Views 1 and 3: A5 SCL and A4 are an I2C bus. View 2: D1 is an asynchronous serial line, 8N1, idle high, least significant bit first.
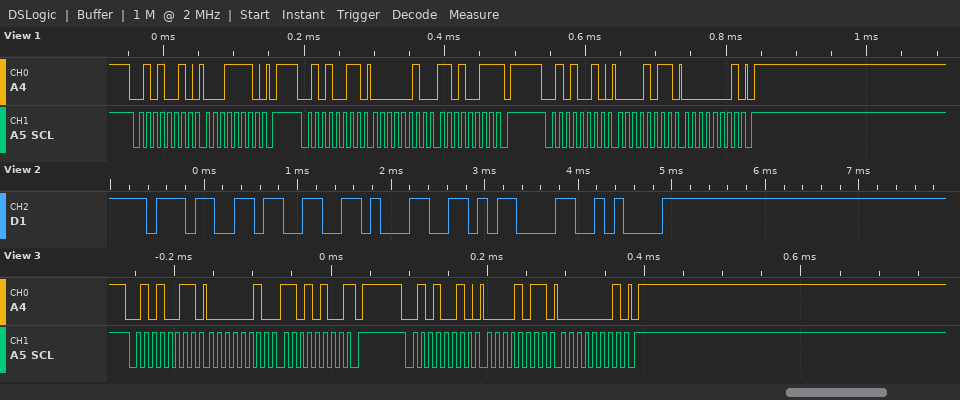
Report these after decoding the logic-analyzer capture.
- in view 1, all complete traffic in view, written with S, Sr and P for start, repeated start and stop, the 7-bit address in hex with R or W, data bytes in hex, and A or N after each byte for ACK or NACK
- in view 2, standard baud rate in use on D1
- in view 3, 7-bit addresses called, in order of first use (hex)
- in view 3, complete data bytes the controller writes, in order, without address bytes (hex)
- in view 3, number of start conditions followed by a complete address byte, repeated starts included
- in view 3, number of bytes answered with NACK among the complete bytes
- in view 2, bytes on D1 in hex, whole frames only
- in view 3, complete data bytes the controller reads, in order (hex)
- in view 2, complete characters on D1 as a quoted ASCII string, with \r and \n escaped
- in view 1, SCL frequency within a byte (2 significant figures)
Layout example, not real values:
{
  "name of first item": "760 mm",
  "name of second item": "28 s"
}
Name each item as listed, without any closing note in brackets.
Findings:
{
  "in view 1, all complete traffic in view, written with S, Sr and P for start, repeated start and stop, the 7-bit address in hex with R or W, data bytes in hex, and A or N after each byte for ACK or NACK": "S 29W A 1E A P S 29R A 02 A D3 N P S 29W A 0B A 01 A P",
  "in view 2, standard baud rate in use on D1": "9600 baud",
  "in view 3, 7-bit addresses called, in order of first use": "0x29",
  "in view 3, complete data bytes the controller writes, in order, without address bytes": "0B 01",
  "in view 3, number of start conditions followed by a complete address byte, repeated starts included": "2",
  "in view 3, number of bytes answered with NACK among the complete bytes": "1",
  "in view 2, bytes on D1 in hex, whole frames only": "37 33 31 0D 0A",
  "in view 3, complete data bytes the controller reads, in order": "02 D4",
  "in view 2, complete characters on D1 as a quoted ASCII string, with \\r and \\n escaped": "\"731\\r\\n\"",
  "in view 1, SCL frequency within a byte": "100 kHz"
}
